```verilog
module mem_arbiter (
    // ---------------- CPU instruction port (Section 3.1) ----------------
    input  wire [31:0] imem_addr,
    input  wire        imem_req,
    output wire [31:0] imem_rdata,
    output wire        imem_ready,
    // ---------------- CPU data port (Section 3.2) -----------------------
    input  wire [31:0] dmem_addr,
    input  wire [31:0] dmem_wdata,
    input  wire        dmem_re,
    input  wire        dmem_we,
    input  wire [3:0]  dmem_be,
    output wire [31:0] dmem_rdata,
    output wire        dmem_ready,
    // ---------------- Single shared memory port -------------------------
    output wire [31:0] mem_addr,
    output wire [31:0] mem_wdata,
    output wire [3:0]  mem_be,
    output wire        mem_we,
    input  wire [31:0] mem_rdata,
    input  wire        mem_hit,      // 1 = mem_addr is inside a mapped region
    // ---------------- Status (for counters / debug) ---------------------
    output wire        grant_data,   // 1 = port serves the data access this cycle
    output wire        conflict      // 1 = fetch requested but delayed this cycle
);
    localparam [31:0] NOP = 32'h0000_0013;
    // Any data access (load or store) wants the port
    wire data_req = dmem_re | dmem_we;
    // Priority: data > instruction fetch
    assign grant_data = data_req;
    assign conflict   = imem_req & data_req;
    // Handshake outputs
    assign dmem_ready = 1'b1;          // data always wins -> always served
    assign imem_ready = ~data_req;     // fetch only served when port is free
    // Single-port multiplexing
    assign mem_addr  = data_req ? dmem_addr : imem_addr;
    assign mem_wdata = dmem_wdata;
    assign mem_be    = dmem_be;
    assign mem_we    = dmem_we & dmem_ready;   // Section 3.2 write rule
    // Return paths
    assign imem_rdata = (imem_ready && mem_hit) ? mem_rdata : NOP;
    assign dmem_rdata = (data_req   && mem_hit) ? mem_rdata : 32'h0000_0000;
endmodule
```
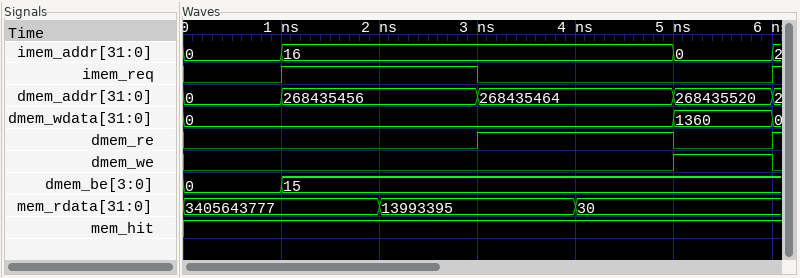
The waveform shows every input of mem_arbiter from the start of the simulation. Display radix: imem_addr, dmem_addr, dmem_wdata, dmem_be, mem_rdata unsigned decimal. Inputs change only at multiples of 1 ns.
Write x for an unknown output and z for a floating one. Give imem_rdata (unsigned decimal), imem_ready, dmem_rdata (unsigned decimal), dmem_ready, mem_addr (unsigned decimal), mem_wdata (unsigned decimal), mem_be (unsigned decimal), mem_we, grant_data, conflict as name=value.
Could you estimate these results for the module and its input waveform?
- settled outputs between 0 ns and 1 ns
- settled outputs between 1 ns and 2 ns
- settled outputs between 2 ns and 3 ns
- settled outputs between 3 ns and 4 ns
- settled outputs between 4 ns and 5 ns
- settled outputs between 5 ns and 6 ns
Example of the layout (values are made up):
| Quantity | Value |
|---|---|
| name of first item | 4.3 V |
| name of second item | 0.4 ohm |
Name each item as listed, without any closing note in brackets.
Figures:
| Quantity | Value |
|---|---|
| settled outputs between 0 ns and 1 ns | imem_rdata=3405643777, imem_ready=1, dmem_rdata=0, dmem_ready=1, mem_addr=0, mem_wdata=0, mem_be=0, mem_we=0, grant_data=0, conflict=0 |
| settled outputs between 1 ns and 2 ns | imem_rdata=3405643777, imem_ready=1, dmem_rdata=0, dmem_ready=1, mem_addr=16, mem_wdata=0, mem_be=15, mem_we=0, grant_data=0, conflict=0 |
| settled outputs between 2 ns and 3 ns | imem_rdata=13993395, imem_ready=1, dmem_rdata=0, dmem_ready=1, mem_addr=16, mem_wdata=0, mem_be=15, mem_we=0, grant_data=0, conflict=0 |
| settled outputs between 3 ns and 4 ns | imem_rdata=19, imem_ready=0, dmem_rdata=13993395, dmem_ready=1, mem_addr=268435464, mem_wdata=0, mem_be=15, mem_we=0, grant_data=1, conflict=0 |
| settled outputs between 4 ns and 5 ns | imem_rdata=19, imem_ready=0, dmem_rdata=30, dmem_ready=1, mem_addr=268435464, mem_wdata=0, mem_be=15, mem_we=0, grant_data=1, conflict=0 |
| settled outputs between 5 ns and 6 ns | imem_rdata=19, imem_ready=0, dmem_rdata=30, dmem_ready=1, mem_addr=268435520, mem_wdata=1360, mem_be=15, mem_we=1, grant_data=1, conflict=0 |
